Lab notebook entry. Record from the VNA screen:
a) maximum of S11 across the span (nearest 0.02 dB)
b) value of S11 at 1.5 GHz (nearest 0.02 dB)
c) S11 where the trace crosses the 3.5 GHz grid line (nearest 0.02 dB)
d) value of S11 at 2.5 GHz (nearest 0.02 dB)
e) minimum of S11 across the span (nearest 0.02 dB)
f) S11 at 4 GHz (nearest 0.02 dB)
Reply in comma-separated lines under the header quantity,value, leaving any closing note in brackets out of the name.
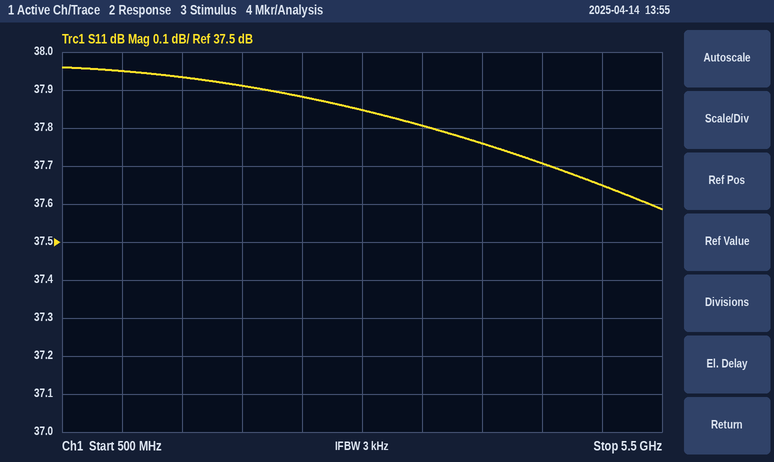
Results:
quantity,value
maximum of S11 across the span,37.96 dB
value of S11 at 1.5 GHz,37.94 dB
S11 where the trace crosses the 3.5 GHz grid line,37.80 dB
value of S11 at 2.5 GHz,37.88 dB
minimum of S11 across the span,37.58 dB
S11 at 4 GHz,37.76 dB
